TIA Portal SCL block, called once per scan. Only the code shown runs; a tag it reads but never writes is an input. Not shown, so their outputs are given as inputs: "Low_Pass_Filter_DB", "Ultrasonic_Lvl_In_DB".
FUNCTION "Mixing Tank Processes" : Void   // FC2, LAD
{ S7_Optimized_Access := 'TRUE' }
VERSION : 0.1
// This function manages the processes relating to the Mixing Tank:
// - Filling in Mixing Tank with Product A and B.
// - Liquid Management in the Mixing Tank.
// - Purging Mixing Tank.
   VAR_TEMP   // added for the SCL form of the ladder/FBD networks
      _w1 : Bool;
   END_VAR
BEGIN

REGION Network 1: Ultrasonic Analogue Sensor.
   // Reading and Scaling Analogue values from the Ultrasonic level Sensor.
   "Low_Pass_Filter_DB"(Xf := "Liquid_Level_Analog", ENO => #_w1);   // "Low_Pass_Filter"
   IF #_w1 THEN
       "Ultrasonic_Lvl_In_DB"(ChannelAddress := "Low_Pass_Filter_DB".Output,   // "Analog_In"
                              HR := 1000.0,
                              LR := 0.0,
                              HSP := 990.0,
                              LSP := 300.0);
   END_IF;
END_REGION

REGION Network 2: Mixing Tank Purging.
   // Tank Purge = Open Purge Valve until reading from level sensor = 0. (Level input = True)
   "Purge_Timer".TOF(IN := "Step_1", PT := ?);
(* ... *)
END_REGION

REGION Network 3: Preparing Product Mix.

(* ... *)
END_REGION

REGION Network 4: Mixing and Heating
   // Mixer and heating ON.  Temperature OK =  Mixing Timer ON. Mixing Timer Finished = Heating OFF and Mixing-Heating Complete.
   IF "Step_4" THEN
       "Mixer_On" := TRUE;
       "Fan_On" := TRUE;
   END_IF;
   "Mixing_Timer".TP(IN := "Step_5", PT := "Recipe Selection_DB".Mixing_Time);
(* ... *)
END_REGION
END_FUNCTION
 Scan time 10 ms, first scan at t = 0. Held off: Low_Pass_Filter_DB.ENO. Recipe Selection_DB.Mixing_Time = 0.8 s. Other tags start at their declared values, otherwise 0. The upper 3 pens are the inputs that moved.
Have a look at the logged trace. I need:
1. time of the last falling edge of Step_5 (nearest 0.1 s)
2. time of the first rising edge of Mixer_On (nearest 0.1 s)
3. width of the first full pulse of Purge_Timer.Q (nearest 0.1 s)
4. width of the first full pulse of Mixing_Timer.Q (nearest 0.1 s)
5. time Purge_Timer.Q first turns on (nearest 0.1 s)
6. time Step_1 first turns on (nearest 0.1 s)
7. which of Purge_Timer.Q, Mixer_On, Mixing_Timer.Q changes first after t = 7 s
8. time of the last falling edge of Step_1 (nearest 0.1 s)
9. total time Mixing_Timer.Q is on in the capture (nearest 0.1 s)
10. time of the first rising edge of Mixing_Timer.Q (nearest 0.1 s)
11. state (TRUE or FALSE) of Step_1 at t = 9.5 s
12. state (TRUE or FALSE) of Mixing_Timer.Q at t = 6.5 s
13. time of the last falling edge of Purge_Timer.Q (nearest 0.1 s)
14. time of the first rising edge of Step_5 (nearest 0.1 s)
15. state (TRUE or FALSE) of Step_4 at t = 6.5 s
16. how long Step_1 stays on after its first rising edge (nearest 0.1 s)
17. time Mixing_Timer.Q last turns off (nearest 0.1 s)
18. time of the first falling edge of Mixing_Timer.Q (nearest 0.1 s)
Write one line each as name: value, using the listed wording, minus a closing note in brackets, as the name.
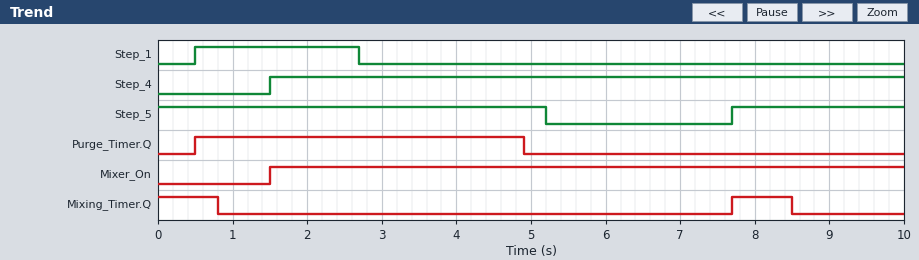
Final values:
time of the last falling edge of Step_5: 5.2 s
time of the first rising edge of Mixer_On: 1.5 s
width of the first full pulse of Purge_Timer.Q: 4.4 s
width of the first full pulse of Mixing_Timer.Q: 0.8 s
time Purge_Timer.Q first turns on: 0.5 s
time Step_1 first turns on: 0.5 s
which of Purge_Timer.Q, Mixer_On, Mixing_Timer.Q changes first after t = 7 s: Mixing_Timer.Q
time of the last falling edge of Step_1: 2.7 s
total time Mixing_Timer.Q is on in the capture: 1.6 s
time of the first rising edge of Mixing_Timer.Q: 7.7 s
state (TRUE or FALSE) of Step_1 at t = 9.5 s: FALSE
state (TRUE or FALSE) of Mixing_Timer.Q at t = 6.5 s: FALSE
time of the last falling edge of Purge_Timer.Q: 4.9 s
time of the first rising edge of Step_5: 7.7 s
state (TRUE or FALSE) of Step_4 at t = 6.5 s: TRUE
how long Step_1 stays on after its first rising edge: 2.2 s
time Mixing_Timer.Q last turns off: 8.5 s
time of the first falling edge of Mixing_Timer.Q: 0.8 s
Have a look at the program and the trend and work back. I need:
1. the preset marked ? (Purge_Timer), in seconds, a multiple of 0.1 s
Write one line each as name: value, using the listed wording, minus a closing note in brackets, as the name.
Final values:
the preset marked ? (Purge_Timer), in seconds, a multiple of 0.1 s: 2.2 s
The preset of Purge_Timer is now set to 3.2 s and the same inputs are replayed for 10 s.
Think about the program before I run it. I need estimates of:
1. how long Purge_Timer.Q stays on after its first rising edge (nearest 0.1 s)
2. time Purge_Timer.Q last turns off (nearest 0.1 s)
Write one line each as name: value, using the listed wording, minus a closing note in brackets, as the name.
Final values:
how long Purge_Timer.Q stays on after its first rising edge: 5.4 s
time Purge_Timer.Q last turns off: 5.9 s
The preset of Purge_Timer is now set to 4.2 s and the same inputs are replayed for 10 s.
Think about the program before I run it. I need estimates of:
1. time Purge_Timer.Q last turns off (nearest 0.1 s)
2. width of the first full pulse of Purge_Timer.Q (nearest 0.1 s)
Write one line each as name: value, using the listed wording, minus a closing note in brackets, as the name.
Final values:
time Purge_Timer.Q last turns off: 6.9 s
width of the first full pulse of Purge_Timer.Q: 6.4 s
